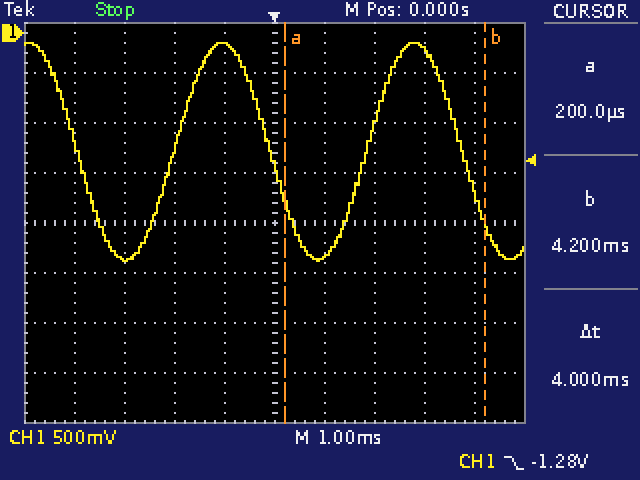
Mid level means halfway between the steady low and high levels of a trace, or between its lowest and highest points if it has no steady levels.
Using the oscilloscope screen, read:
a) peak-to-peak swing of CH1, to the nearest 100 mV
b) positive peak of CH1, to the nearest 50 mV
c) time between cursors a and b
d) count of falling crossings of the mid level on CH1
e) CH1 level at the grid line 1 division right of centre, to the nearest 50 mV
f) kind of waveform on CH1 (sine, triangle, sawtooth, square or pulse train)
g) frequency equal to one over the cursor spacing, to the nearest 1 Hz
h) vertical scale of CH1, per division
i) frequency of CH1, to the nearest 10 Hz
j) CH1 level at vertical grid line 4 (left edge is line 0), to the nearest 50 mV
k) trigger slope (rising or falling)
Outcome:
2.20 V
-100 mV
4 ms
3
-2.25 V
sine
250 Hz
500 mV
260 Hz
-100 mV
falling
